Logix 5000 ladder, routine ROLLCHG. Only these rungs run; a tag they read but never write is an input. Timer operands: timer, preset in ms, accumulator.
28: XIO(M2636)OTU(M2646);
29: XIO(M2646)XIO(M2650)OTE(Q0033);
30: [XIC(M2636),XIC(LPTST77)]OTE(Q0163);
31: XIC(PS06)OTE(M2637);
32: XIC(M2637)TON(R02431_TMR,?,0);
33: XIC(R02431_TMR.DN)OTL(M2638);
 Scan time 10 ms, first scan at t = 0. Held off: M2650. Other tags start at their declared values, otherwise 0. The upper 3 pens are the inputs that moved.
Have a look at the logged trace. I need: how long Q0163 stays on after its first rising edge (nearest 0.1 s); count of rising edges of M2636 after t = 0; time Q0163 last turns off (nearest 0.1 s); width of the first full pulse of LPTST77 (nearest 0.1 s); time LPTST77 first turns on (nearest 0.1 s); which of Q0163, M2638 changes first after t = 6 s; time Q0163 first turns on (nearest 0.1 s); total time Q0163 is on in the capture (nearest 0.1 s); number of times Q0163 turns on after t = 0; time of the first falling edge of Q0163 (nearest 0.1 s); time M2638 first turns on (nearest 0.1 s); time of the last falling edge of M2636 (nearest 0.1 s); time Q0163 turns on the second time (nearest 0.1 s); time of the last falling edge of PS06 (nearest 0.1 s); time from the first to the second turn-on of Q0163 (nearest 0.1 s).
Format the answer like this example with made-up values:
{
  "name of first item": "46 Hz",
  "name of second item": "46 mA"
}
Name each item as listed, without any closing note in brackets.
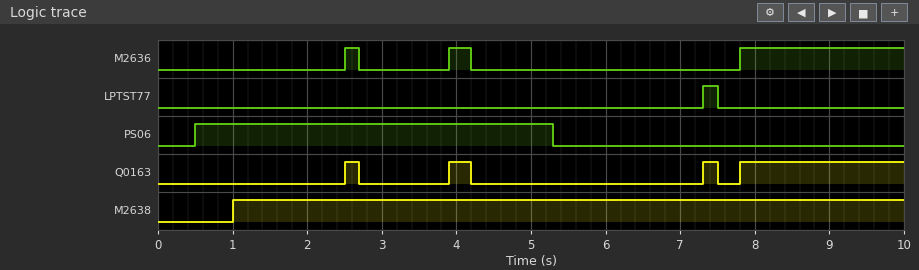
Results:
{
  "how long Q0163 stays on after its first rising edge": "0.2 s",
  "count of rising edges of M2636 after t = 0": "3",
  "time Q0163 last turns off": "7.5 s",
  "width of the first full pulse of LPTST77": "0.2 s",
  "time LPTST77 first turns on": "7.3 s",
  "which of Q0163, M2638 changes first after t = 6 s": "Q0163",
  "time Q0163 first turns on": "2.5 s",
  "total time Q0163 is on in the capture": "2.9 s",
  "number of times Q0163 turns on after t = 0": "4",
  "time of the first falling edge of Q0163": "2.7 s",
  "time M2638 first turns on": "1.0 s",
  "time of the last falling edge of M2636": "4.2 s",
  "time Q0163 turns on the second time": "3.9 s",
  "time of the last falling edge of PS06": "5.3 s",
  "time from the first to the second turn-on of Q0163": "1.4 s"
}
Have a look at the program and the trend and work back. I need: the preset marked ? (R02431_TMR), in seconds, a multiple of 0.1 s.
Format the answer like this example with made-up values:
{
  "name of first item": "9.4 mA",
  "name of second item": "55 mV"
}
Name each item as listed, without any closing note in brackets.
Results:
{
  "the preset marked ? (R02431_TMR), in seconds, a multiple of 0.1 s": "0.5 s"
}
